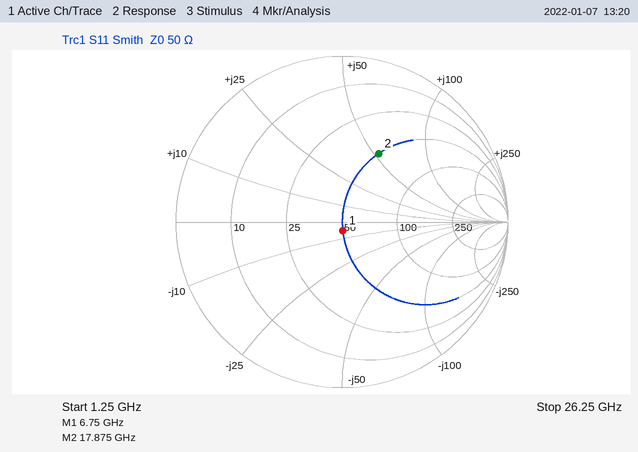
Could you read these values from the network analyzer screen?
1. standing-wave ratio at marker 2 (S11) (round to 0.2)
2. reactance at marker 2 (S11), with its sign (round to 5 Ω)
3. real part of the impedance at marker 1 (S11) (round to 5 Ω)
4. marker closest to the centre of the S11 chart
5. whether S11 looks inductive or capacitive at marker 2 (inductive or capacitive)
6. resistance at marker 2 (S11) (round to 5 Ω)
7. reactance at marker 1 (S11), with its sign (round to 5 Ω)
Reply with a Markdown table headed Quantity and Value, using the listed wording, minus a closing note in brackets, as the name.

| Quantity | Value |
|---|---|
| standing-wave ratio at marker 2 (S11) | 2.8 |
| reactance at marker 2 (S11), with its sign | +55 Ω |
| real part of the impedance at marker 1 (S11) | 50 Ω |
| marker closest to the centre of the S11 chart | marker 1 |
| whether S11 looks inductive or capacitive at marker 2 | inductive |
| resistance at marker 2 (S11) | 50 Ω |
| reactance at marker 1 (S11), with its sign | -5 Ω |
